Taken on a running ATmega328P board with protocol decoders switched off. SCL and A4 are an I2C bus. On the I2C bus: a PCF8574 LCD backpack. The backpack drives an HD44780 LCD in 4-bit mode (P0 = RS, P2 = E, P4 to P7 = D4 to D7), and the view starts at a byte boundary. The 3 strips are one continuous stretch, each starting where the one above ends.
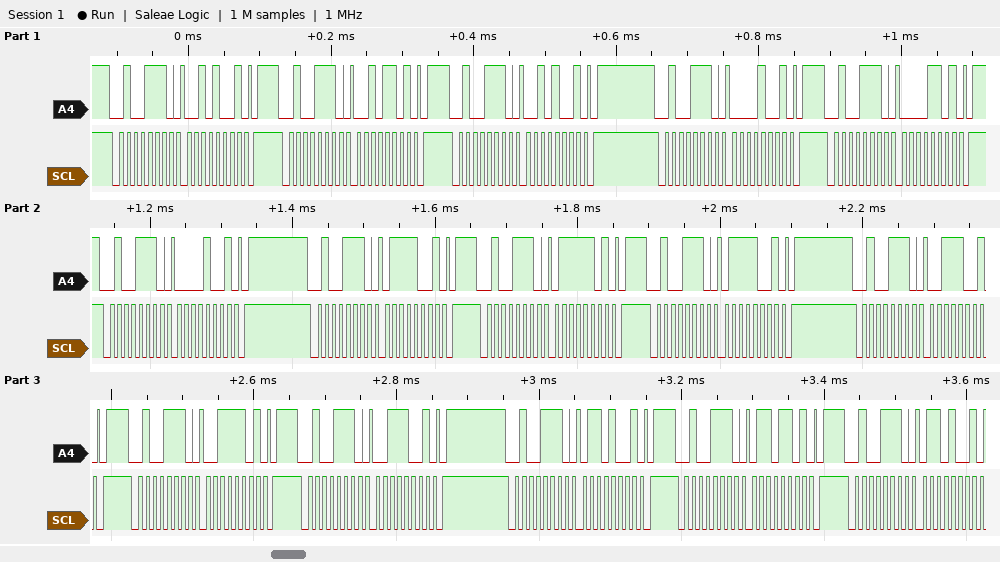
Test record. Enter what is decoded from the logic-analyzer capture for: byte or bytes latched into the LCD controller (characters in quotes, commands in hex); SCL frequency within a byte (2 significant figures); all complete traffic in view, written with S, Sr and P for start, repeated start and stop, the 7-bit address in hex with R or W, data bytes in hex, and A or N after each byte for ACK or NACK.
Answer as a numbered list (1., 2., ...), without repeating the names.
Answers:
1. ' ' 's'
2. 100 kHz
3. S 27W A 29 A P S 27W A 2D A P S 27W A 29 A P S 27W A 09 A P S 27W A 0D A P S 27W A 09 A P S 27W A 79 A P S 27W A 7D A P S 27W A 79 A P S 27W A 39 A P S 27W A 3D A P S 27W A 39 A P S 27W A 69 A P S 27W A 6D A P S 27W A 69 A
